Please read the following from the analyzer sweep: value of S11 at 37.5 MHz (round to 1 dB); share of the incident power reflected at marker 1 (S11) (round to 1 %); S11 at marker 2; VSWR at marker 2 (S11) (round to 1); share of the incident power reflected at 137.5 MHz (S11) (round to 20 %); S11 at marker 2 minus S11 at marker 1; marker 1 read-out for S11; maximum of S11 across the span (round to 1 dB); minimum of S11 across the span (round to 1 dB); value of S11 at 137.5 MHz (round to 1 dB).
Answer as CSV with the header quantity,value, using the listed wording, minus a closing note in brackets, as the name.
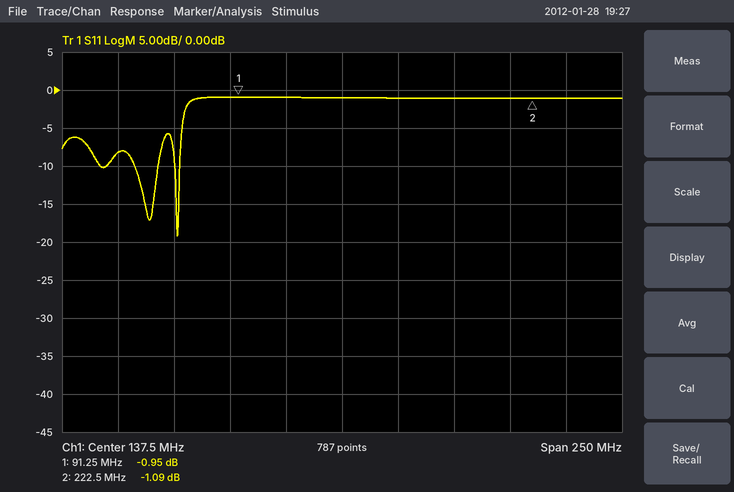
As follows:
quantity,value
value of S11 at 37.5 MHz,-8 dB
share of the incident power reflected at marker 1 (S11),80 %
S11 at marker 2,-1.09 dB
VSWR at marker 2 (S11),16
share of the incident power reflected at 137.5 MHz (S11),80 %
S11 at marker 2 minus S11 at marker 1,-0.14 dB
marker 1 read-out for S11,-0.95 dB
maximum of S11 across the span,-1 dB
minimum of S11 across the span,-19 dB
value of S11 at 137.5 MHz,-1 dB
